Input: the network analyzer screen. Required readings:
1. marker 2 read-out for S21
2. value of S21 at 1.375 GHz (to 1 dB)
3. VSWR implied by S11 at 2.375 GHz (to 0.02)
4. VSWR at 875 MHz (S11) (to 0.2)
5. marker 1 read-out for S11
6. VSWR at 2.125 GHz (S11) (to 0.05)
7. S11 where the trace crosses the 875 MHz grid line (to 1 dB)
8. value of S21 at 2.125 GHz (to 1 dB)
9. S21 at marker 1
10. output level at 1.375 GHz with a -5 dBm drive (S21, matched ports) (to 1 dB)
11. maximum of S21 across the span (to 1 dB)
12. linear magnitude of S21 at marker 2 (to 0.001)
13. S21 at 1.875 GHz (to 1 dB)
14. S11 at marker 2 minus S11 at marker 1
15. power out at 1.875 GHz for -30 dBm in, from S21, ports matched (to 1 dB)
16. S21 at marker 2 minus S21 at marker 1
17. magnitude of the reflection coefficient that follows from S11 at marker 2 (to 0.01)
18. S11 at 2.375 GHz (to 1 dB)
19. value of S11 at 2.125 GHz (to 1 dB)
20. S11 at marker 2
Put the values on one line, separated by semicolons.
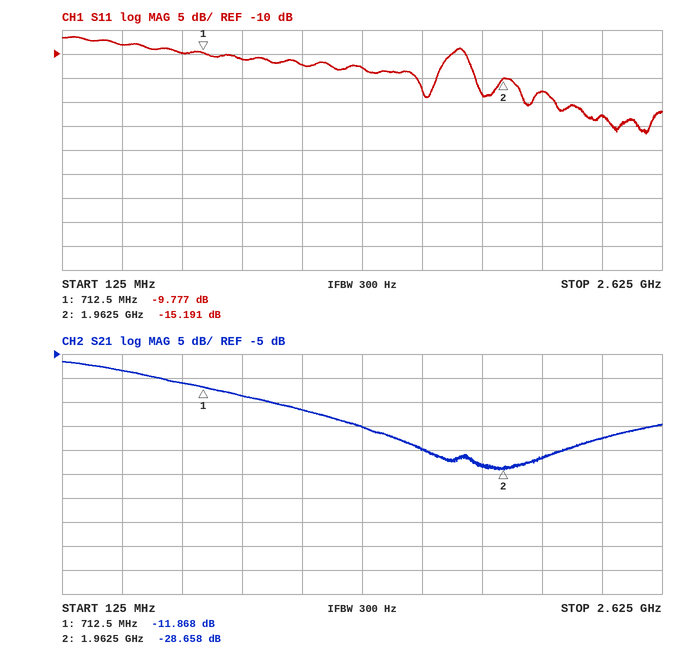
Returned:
-28.658 dB; -20 dB; 1.16; 1.8; -9.777 dB; 1.30; -11 dB; -27 dB; -11.868 dB; -25 dBm; -7 dB; 0.037; -28 dB; -5.414 dB; -58 dBm; -16.790 dB; 0.17; -23 dB; -18 dB; -15.191 dB
